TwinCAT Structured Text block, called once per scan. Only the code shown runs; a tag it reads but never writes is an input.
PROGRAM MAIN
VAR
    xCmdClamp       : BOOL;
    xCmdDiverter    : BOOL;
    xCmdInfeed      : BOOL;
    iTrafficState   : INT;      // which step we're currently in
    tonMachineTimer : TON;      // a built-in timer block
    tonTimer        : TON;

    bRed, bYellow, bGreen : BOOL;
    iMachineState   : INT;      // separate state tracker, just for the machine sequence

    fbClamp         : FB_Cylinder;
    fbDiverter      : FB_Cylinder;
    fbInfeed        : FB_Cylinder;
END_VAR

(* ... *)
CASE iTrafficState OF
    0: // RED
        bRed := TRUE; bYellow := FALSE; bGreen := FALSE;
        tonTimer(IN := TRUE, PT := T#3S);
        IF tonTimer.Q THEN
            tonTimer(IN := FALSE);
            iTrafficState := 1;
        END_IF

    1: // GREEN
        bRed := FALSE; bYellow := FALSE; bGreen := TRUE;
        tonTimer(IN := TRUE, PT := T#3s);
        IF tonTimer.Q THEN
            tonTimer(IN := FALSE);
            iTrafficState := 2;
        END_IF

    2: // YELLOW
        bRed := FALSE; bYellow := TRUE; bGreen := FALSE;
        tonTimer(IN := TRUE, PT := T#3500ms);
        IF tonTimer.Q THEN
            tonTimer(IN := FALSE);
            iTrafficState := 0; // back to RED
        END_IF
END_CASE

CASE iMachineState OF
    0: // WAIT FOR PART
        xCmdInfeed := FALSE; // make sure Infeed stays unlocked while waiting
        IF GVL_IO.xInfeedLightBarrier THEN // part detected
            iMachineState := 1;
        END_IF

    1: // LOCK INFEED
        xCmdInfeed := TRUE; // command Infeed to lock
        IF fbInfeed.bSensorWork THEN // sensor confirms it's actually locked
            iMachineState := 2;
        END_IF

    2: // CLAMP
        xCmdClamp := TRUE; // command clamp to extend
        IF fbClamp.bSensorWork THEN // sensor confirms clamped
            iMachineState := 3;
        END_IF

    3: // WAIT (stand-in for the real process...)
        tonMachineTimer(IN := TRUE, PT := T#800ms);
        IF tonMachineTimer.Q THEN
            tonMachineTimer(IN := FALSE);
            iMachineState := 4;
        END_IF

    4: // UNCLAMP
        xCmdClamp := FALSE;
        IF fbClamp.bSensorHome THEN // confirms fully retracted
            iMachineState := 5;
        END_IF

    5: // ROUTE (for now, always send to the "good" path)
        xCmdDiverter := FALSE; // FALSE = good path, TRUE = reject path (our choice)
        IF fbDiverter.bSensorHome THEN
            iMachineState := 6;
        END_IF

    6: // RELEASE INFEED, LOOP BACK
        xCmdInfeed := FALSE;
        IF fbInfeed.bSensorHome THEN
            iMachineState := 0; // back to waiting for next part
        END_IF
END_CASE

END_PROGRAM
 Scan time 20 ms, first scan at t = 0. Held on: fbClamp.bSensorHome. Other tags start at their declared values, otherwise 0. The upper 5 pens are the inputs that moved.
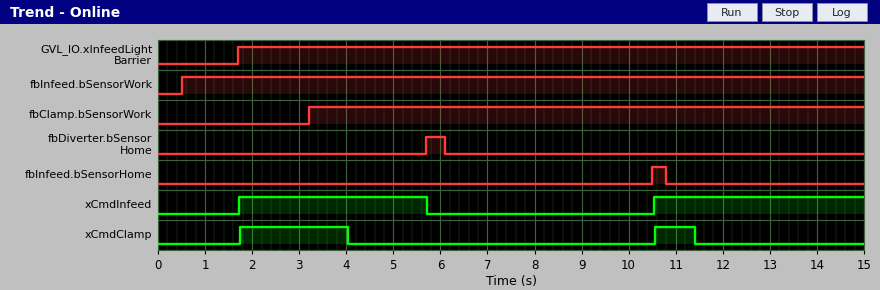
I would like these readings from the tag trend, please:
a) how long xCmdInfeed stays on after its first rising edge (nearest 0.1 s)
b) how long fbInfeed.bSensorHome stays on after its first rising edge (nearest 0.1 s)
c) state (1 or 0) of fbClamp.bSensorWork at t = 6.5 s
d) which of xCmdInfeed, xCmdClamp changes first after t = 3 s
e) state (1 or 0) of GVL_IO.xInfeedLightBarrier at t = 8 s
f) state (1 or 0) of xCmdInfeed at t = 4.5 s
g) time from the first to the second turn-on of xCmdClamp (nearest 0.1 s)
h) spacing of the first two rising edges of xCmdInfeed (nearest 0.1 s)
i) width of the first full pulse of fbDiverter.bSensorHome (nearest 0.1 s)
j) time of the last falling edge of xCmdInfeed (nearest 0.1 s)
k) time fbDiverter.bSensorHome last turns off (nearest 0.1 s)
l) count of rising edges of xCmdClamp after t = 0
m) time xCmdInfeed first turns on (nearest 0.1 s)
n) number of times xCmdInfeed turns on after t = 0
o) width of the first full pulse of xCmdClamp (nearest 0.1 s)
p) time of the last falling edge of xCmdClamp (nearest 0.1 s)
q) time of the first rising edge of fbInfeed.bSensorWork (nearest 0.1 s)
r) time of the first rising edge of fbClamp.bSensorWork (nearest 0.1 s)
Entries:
4.0 s
0.3 s
1
xCmdClamp
1
1
8.8 s
8.8 s
0.4 s
5.7 s
6.1 s
2
1.7 s
2
2.3 s
11.4 s
0.5 s
3.2 s
